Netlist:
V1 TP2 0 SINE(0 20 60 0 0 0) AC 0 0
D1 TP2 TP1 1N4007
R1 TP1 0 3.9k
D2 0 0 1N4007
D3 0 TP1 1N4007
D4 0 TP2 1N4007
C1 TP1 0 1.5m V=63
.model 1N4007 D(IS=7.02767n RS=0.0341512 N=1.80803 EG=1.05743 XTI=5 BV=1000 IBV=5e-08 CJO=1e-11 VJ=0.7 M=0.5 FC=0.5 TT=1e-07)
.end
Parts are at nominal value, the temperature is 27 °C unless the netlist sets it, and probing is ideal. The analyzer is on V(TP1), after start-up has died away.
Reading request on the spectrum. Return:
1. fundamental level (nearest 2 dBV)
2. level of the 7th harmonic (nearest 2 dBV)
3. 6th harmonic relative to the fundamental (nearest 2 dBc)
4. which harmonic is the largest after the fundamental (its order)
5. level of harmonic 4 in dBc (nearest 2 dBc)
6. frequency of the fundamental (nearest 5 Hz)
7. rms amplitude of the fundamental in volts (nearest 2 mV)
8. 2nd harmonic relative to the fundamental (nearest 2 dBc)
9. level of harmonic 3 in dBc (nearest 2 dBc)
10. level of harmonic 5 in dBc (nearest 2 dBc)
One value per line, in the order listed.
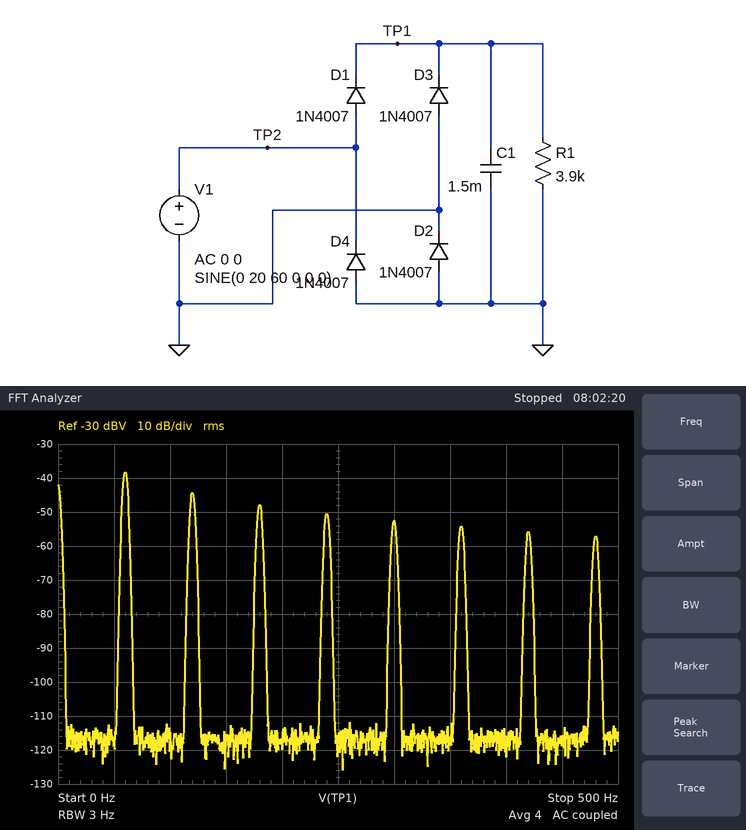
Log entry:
-38 dBV
-56 dBV
-16 dBc
2
-12 dBc
60 Hz
12 mV
-6 dBc
-10 dBc
-14 dBc
